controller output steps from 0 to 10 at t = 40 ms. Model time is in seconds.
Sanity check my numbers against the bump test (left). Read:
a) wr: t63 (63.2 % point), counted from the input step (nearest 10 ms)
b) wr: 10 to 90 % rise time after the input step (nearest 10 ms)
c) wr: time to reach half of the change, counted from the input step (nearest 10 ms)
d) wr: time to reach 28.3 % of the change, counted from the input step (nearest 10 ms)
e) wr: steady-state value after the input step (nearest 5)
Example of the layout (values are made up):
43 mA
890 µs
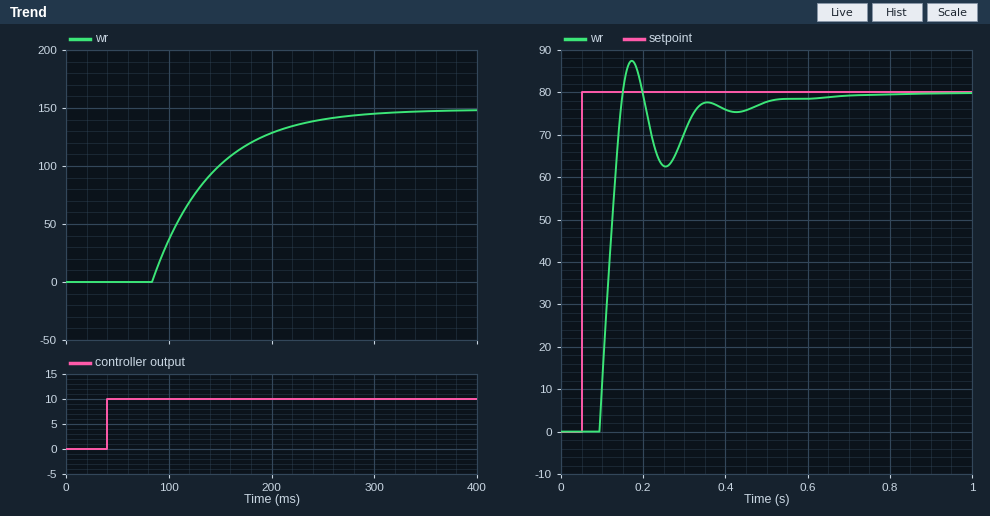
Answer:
100 ms
130 ms
80 ms
60 ms
150
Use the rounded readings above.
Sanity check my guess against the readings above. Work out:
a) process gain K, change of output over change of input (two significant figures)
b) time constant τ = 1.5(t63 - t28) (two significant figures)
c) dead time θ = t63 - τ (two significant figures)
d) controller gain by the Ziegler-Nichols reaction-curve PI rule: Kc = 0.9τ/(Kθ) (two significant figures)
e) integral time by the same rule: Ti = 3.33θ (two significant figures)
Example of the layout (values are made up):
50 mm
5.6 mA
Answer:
15
60 ms
40 ms
0.090
130 ms
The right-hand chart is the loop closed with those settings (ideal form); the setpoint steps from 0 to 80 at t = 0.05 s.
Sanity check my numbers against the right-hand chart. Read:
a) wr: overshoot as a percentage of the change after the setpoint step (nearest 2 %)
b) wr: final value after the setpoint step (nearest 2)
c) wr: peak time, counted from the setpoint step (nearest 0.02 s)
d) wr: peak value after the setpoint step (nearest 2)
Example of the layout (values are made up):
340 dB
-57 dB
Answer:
10 %
80
0.12 s
88
